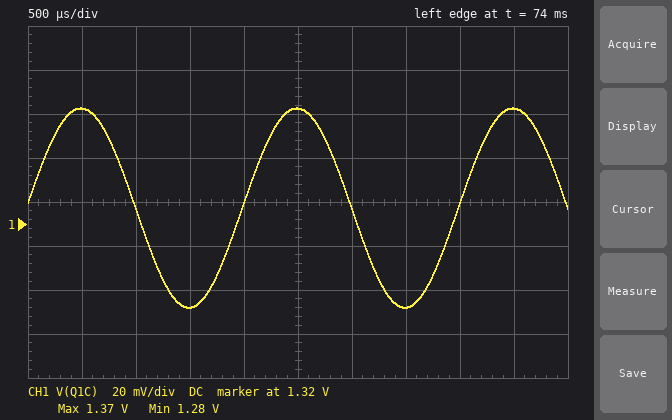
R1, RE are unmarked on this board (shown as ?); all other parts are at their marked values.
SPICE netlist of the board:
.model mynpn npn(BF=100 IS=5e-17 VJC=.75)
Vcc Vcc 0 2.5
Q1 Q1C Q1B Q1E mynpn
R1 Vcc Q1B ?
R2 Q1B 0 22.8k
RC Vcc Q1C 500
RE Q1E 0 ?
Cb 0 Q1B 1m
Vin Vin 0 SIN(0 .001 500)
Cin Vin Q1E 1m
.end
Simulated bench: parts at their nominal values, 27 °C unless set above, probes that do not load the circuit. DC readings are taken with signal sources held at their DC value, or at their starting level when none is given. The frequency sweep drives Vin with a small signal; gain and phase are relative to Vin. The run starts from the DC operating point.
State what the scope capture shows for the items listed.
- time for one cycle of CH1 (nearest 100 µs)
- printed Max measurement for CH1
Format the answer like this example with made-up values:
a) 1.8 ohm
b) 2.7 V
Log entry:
a) 2.0 ms
b) 1.37 V
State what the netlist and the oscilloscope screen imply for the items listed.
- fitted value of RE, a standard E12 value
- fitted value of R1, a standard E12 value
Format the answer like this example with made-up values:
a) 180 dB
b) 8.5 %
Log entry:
a) 270 Ω
b) 12 kΩ
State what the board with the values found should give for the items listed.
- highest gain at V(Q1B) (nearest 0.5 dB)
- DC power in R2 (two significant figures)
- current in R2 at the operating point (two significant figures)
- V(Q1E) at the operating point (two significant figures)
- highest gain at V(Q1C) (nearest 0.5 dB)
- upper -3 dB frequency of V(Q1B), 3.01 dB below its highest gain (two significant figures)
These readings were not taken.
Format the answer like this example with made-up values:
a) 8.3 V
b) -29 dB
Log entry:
a) -40.5 dB
b) 93 µW
c) 64 µA
d) 640 mV
e) 33.0 dB
f) 15 Hz
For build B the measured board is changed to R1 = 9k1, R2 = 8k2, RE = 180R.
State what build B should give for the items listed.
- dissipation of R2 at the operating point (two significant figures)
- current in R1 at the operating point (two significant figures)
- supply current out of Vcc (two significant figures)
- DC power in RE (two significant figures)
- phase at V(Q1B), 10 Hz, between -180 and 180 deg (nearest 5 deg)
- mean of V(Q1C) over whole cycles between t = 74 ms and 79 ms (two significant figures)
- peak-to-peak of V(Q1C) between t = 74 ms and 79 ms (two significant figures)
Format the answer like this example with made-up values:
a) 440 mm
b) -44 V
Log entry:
a) 150 µW
b) 150 µA
c) 1.8 mA
d) 520 µW
e) -40 deg
f) 1.7 V
g) 65 mV
